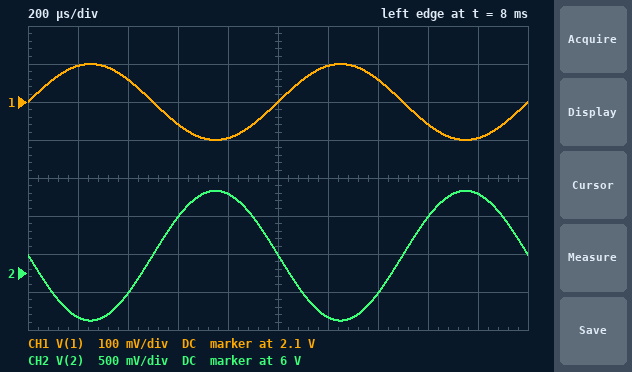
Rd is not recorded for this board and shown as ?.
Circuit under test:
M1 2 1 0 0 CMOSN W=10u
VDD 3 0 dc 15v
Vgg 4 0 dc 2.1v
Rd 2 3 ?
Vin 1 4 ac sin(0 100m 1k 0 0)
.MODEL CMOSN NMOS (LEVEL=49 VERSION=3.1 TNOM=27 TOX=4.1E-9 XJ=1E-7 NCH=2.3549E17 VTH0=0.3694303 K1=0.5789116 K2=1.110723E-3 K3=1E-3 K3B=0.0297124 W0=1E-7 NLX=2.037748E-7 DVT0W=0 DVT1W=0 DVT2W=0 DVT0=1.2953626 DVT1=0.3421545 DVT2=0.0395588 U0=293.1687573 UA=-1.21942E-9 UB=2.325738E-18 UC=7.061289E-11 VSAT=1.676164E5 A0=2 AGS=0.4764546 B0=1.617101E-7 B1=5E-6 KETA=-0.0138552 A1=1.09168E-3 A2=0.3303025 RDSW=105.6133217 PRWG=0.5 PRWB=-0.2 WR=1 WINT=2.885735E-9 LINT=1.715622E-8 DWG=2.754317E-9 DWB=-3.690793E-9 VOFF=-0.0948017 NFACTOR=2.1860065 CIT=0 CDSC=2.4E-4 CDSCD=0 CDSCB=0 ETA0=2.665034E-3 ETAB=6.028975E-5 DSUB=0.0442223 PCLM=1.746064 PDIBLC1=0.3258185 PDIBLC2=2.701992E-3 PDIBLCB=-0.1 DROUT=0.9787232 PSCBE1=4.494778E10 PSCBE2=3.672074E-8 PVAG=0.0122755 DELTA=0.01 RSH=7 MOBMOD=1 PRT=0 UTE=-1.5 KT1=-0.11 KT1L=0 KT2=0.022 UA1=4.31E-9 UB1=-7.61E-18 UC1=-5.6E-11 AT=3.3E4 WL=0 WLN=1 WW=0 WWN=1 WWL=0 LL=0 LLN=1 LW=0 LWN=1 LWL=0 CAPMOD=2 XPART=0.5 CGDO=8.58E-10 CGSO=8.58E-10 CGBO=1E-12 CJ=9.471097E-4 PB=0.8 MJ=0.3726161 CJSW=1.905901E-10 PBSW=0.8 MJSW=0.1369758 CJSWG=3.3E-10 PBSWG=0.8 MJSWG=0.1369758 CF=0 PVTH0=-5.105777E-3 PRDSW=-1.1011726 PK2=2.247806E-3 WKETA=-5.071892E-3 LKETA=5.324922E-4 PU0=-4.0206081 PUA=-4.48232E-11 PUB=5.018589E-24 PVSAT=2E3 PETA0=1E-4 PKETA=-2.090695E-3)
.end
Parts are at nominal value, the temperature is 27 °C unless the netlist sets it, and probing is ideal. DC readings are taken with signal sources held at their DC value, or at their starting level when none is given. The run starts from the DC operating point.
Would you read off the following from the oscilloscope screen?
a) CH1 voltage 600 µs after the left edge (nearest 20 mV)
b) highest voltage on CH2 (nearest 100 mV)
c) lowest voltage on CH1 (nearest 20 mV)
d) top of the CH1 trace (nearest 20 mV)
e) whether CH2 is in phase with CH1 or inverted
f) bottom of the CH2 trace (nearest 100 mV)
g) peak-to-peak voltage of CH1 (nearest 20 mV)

2.04 V
7.1 V
2.00 V
2.20 V
inverted
5.4 V
200 mV
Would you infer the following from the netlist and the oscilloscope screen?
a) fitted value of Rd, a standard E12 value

15 kΩ
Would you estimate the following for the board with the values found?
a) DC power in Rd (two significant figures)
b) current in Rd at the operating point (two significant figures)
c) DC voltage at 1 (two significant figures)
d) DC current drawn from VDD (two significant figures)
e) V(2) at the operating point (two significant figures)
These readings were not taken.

5.1 mW
580 µA
2.1 V
580 µA
6.2 V
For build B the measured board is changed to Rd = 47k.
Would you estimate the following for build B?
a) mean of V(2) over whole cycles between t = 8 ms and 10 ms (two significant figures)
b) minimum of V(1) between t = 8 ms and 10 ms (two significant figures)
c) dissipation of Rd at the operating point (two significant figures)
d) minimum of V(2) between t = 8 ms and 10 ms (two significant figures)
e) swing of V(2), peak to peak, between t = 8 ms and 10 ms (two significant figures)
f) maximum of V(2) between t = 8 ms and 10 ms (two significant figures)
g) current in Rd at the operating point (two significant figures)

500 mV
2.0 V
4.5 mW
480 mV
46 mV
520 mV
310 µA
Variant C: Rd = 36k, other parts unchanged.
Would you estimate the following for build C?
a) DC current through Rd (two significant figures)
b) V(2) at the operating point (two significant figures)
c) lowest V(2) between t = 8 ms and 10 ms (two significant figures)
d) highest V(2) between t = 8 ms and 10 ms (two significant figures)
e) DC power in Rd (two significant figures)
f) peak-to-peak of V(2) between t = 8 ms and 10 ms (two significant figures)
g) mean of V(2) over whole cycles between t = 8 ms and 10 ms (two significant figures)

400 µA
690 mV
660 mV
750 mV
5.7 mW
88 mV
700 mV
